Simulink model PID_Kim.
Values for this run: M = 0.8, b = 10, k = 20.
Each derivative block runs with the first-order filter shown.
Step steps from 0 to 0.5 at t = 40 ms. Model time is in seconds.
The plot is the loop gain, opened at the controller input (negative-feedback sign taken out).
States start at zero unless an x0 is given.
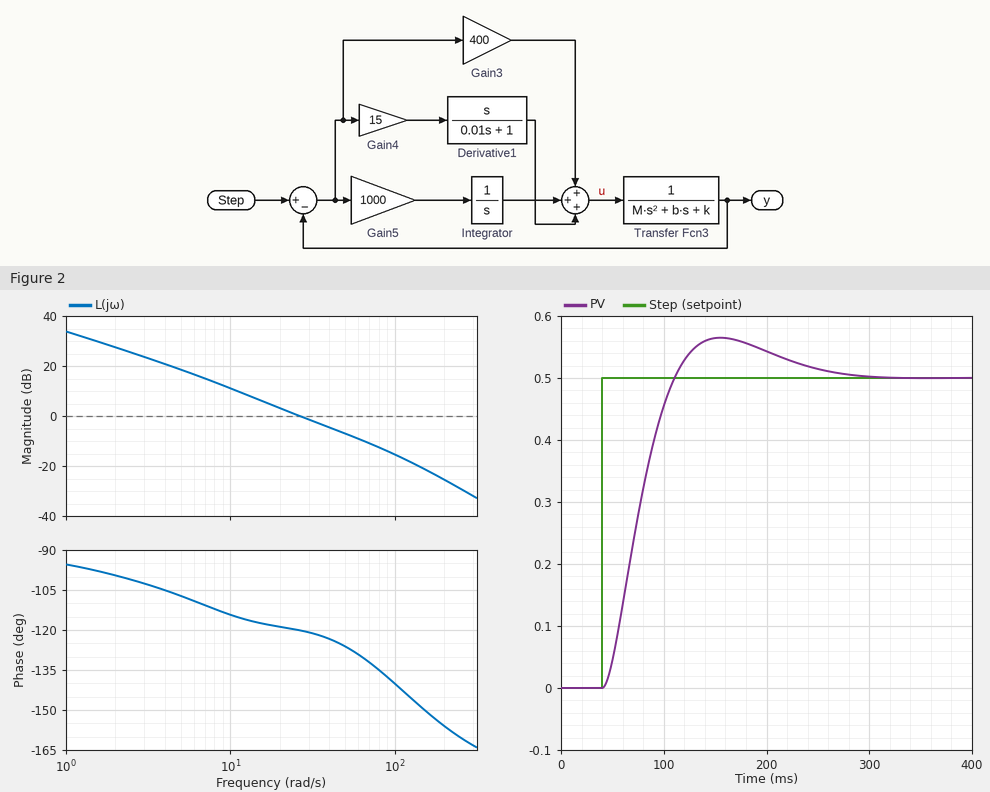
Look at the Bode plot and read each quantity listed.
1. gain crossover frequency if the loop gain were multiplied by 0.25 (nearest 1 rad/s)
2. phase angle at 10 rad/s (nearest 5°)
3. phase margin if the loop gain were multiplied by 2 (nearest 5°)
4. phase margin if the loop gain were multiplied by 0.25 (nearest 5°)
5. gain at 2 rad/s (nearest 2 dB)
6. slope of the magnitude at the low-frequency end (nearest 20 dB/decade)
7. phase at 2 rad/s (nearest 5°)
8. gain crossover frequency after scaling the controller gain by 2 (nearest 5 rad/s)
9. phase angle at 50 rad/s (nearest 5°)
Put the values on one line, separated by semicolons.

9 rad/s; -115°; 55°; 65°; 28 dB; -20 dB/decade; -100°; 45 rad/s; -125°
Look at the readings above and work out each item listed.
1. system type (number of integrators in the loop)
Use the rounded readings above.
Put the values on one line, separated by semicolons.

1
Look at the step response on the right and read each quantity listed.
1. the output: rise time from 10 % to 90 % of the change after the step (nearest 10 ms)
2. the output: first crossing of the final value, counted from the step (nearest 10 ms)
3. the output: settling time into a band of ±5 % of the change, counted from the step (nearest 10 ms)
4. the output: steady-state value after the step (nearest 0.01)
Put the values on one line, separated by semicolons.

50 ms; 70 ms; 190 ms; 0.50
